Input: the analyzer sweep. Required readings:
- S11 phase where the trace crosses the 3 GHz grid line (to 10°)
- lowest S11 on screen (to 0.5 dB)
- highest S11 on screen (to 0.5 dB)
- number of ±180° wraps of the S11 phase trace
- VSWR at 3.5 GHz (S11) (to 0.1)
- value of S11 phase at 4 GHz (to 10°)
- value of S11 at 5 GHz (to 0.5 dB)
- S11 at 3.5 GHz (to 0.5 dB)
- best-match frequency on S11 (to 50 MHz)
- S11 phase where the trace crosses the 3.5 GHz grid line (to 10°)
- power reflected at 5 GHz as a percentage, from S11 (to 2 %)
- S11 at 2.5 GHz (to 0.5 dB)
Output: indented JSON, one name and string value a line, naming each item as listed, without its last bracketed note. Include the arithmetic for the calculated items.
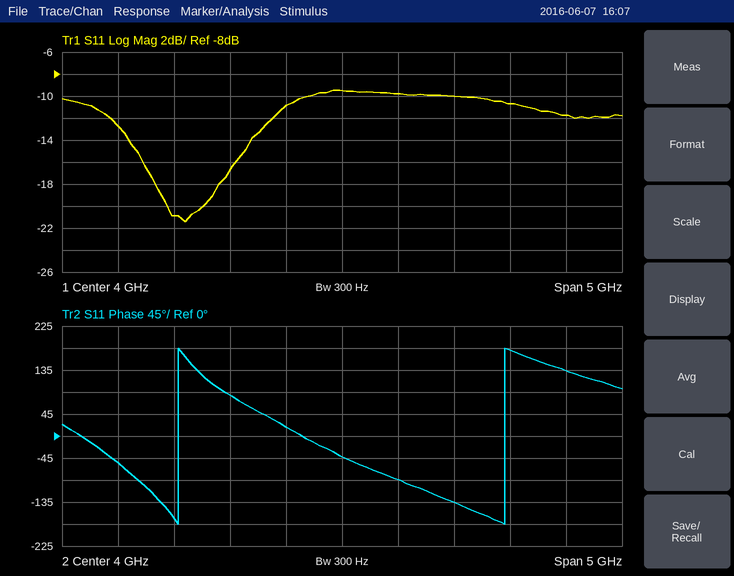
{
  "S11 phase where the trace crosses the 3 GHz grid line": "80°",
  "lowest S11 on screen": "-21.5 dB",
  "highest S11 on screen": "-9.5 dB",
  "number of ±180° wraps of the S11 phase trace": "2",
  "VSWR at 3.5 GHz (S11)": "|Γ| = 10^(-11/20) = 0.2818; VSWR = (1 + 0.2818)/(1 − 0.2818) ≈ 1.8",
  "value of S11 phase at 4 GHz": "-40°",
  "value of S11 at 5 GHz": "-10.0 dB",
  "S11 at 3.5 GHz": "-11.0 dB",
  "best-match frequency on S11": "2.60 GHz",
  "S11 phase where the trace crosses the 3.5 GHz grid line": "20°",
  "power reflected at 5 GHz as a percentage, from S11": "10^(-10/10) ≈ 10 %",
  "S11 at 2.5 GHz": "-21.0 dB"
}
